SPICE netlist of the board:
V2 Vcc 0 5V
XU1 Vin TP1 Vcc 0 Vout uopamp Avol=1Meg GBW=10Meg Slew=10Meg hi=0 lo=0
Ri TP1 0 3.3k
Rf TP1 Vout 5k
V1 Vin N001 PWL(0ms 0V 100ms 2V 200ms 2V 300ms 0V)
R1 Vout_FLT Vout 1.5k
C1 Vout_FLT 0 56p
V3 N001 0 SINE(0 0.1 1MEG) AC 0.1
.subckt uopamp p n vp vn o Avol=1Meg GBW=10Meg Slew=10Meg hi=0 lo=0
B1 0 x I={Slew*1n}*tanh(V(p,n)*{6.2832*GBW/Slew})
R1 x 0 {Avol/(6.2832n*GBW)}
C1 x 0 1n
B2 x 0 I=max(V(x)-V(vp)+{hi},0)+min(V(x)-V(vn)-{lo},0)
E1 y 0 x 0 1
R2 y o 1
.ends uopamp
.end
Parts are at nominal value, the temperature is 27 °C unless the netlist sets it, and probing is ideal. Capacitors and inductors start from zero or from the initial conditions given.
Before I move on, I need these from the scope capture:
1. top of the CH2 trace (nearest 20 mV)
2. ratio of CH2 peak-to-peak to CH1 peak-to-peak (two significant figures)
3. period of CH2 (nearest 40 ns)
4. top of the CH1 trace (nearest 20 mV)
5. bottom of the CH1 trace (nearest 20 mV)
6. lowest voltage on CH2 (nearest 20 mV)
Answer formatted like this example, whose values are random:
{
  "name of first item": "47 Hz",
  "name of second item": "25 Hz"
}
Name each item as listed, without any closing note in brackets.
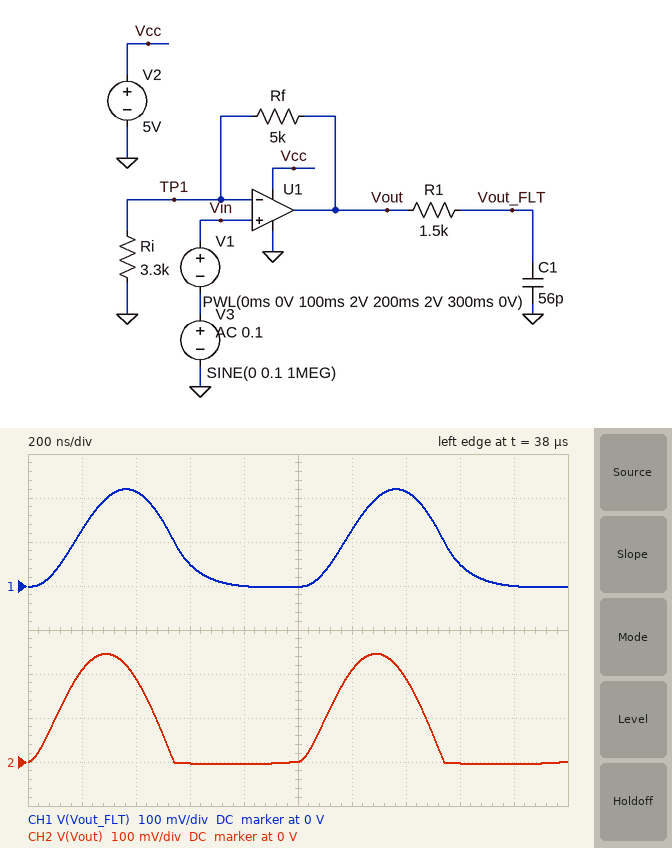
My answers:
{
  "top of the CH2 trace": "240 mV",
  "ratio of CH2 peak-to-peak to CH1 peak-to-peak": "1.1",
  "period of CH2": "1.00 µs",
  "top of the CH1 trace": "220 mV",
  "bottom of the CH1 trace": "0 V",
  "lowest voltage on CH2": "0 V"
}
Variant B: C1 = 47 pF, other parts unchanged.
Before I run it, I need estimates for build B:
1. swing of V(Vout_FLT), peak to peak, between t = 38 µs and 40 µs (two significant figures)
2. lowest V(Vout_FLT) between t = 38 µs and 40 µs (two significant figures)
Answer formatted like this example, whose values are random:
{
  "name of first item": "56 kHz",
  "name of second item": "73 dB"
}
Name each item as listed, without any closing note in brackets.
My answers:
{
  "swing of V(Vout_FLT), peak to peak, between t = 38 µs and 40 µs": "230 mV",
  "lowest V(Vout_FLT) between t = 38 µs and 40 µs": "-4.0 mV"
}
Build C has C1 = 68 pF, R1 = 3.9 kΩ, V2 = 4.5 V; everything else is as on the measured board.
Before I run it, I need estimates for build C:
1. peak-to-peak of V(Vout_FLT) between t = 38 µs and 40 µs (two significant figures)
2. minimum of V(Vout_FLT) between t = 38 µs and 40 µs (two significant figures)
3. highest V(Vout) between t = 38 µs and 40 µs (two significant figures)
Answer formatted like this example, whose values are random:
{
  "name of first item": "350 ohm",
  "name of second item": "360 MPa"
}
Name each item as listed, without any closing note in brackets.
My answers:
{
  "peak-to-peak of V(Vout_FLT) between t = 38 µs and 40 µs": "140 mV",
  "minimum of V(Vout_FLT) between t = 38 µs and 40 µs": "18 mV",
  "highest V(Vout) between t = 38 µs and 40 µs": "250 mV"
}
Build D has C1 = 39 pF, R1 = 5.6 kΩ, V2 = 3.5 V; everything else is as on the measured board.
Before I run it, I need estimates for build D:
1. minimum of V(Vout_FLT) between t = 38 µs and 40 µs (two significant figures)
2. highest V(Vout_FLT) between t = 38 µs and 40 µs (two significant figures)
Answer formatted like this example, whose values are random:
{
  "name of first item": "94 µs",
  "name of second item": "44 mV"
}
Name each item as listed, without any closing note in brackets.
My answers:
{
  "minimum of V(Vout_FLT) between t = 38 µs and 40 µs": "12 mV",
  "highest V(Vout_FLT) between t = 38 µs and 40 µs": "170 mV"
}
